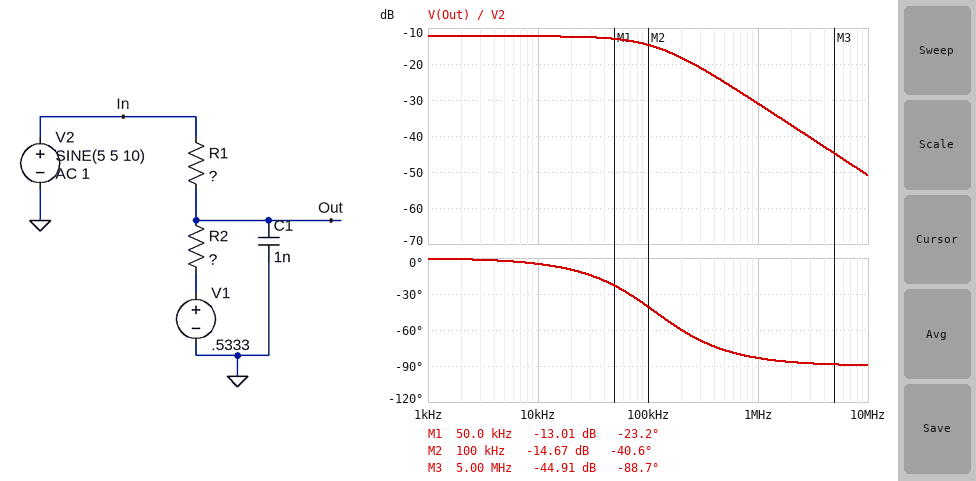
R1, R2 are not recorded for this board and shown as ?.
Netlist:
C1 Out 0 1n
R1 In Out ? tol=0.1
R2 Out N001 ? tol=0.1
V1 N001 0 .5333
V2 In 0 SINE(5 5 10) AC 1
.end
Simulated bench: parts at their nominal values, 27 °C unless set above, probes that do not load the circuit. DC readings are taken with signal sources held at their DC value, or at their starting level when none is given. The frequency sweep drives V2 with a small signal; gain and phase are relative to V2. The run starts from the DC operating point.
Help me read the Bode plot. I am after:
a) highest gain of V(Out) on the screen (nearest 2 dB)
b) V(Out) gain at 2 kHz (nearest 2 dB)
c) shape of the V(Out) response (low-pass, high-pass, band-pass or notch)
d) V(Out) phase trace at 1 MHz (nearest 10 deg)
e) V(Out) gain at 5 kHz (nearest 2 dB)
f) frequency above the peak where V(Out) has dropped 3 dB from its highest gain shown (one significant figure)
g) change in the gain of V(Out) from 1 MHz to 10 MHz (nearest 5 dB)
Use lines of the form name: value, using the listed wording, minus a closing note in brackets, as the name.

highest gain of V(Out) on the screen: -12 dB
V(Out) gain at 2 kHz: -12 dB
shape of the V(Out) response: low-pass
V(Out) phase trace at 1 MHz: -80 deg
V(Out) gain at 5 kHz: -12 dB
frequency above the peak where V(Out) has dropped 3 dB from its highest gain shown: 100 kHz
change in the gain of V(Out) from 1 MHz to 10 MHz: -20 dB
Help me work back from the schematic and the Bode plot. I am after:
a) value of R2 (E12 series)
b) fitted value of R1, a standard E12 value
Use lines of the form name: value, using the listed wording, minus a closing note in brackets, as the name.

value of R2: 1.8 kΩ
fitted value of R1, a standard E12 value: 5.6 kΩ
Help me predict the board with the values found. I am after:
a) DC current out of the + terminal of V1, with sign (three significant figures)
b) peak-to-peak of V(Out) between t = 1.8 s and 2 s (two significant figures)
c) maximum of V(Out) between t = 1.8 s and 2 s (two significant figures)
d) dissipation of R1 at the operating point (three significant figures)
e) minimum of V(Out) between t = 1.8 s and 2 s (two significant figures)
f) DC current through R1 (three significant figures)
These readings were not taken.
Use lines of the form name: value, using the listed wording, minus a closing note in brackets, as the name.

DC current out of the + terminal of V1, with sign: -604 µA
peak-to-peak of V(Out) between t = 1.8 s and 2 s: 2.4 V
maximum of V(Out) between t = 1.8 s and 2 s: 2.8 V
dissipation of R1 at the operating point: 2.04 mW
minimum of V(Out) between t = 1.8 s and 2 s: 400 mV
DC current through R1: 604 µA
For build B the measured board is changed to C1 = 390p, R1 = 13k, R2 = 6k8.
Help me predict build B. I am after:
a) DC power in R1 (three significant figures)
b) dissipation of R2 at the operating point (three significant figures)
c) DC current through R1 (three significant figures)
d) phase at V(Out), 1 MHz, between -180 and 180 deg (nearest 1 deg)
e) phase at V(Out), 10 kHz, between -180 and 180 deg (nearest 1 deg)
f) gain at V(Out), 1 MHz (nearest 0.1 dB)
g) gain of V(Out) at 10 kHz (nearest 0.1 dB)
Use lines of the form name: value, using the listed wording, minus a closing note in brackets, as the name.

DC power in R1: 662 µW
dissipation of R2 at the operating point: 346 µW
DC current through R1: 226 µA
phase at V(Out), 1 MHz, between -180 and 180 deg: -85 deg
phase at V(Out), 10 kHz, between -180 and 180 deg: -6 deg
gain at V(Out), 1 MHz: -30.1 dB
gain of V(Out) at 10 kHz: -9.3 dB
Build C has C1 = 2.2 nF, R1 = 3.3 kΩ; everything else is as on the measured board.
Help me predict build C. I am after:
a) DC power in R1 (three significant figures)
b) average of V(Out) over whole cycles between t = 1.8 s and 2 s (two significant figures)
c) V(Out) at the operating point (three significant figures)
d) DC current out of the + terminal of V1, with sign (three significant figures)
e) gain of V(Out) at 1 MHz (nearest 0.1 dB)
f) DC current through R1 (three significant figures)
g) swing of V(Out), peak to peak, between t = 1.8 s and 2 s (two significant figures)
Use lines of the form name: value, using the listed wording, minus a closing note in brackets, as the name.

DC power in R1: 2.53 mW
average of V(Out) over whole cycles between t = 1.8 s and 2 s: 2.1 V
V(Out) at the operating point: 2.11 V
DC current out of the + terminal of V1, with sign: -876 µA
gain of V(Out) at 1 MHz: -33.2 dB
DC current through R1: 876 µA
swing of V(Out), peak to peak, between t = 1.8 s and 2 s: 3.5 V
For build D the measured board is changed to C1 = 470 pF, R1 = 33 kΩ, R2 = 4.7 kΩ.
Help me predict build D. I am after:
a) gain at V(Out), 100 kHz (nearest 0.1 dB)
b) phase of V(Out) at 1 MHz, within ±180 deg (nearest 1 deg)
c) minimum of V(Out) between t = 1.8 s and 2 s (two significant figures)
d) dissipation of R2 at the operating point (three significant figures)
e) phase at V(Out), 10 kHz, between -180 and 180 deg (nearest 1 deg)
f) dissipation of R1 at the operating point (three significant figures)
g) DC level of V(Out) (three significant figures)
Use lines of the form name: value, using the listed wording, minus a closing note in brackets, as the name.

gain at V(Out), 100 kHz: -22.0 dB
phase of V(Out) at 1 MHz, within ±180 deg: -85 deg
minimum of V(Out) between t = 1.8 s and 2 s: 470 mV
dissipation of R2 at the operating point: 66.0 µW
phase at V(Out), 10 kHz, between -180 and 180 deg: -7 deg
dissipation of R1 at the operating point: 463 µW
DC level of V(Out): 1.09 V
